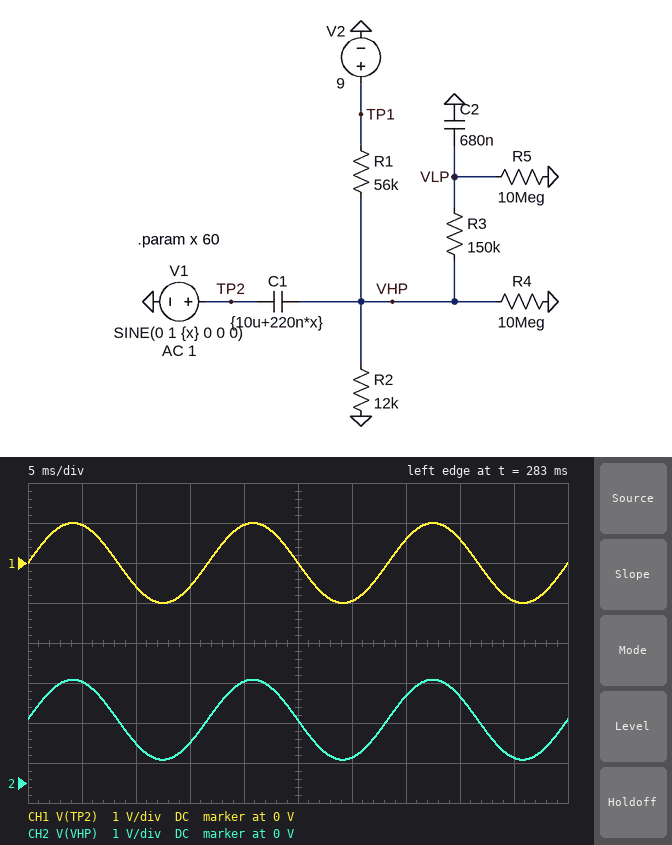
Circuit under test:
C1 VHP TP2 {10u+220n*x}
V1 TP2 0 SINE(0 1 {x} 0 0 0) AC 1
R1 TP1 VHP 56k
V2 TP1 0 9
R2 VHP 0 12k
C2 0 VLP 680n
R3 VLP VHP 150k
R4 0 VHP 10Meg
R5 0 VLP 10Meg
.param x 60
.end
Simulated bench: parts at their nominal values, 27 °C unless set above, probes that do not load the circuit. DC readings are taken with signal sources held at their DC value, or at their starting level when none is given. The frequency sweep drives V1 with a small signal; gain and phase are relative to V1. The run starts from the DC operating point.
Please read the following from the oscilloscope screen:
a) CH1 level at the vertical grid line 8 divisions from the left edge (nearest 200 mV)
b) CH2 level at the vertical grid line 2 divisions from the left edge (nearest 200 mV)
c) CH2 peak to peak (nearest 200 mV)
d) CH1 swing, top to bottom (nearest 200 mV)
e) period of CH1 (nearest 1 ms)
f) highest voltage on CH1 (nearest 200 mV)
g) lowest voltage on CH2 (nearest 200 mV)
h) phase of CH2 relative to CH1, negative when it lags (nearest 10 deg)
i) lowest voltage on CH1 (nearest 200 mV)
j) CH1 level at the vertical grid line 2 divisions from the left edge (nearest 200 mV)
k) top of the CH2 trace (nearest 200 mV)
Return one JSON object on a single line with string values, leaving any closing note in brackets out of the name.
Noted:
{"CH1 level at the vertical grid line 8 divisions from the left edge": "600 mV", "CH2 level at the vertical grid line 2 divisions from the left edge": "1.0 V", "CH2 peak to peak": "2.0 V", "CH1 swing, top to bottom": "2.0 V", "period of CH1": "17 ms", "highest voltage on CH1": "1.0 V", "lowest voltage on CH2": "600 mV", "phase of CH2 relative to CH1, negative when it lags": "0 deg", "lowest voltage on CH1": "-1.0 V", "CH1 level at the vertical grid line 2 divisions from the left edge": "-600 mV", "top of the CH2 trace": "2.6 V"}
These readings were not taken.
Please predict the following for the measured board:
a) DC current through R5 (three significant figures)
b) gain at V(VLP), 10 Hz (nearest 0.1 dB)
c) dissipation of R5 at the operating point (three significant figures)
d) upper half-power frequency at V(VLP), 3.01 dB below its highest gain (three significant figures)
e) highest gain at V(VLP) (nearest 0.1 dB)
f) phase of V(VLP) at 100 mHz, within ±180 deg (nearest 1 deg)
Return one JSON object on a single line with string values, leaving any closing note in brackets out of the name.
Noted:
{"DC current through R5": "156 nA", "gain at V(VLP), 10 Hz": "-16.3 dB", "dissipation of R5 at the operating point": "244 nW", "upper half-power frequency at V(VLP), 3.01 dB below its highest gain": "2.73 Hz", "highest gain at V(VLP)": "-3.5 dB", "phase of V(VLP) at 100 mHz, within ±180 deg": "78 deg"}
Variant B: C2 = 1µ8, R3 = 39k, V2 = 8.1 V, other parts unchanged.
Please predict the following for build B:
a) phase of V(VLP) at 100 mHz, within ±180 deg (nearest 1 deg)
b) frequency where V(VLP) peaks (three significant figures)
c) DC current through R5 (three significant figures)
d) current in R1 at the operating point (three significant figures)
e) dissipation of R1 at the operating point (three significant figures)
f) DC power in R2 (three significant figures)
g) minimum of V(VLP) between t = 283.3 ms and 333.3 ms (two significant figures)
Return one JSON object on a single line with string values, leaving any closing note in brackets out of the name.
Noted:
{"phase of V(VLP) at 100 mHz, within ±180 deg": "79 deg", "frequency where V(VLP) peaks": "1.26 Hz", "DC current through R5": "142 nA", "current in R1 at the operating point": "119 µA", "dissipation of R1 at the operating point": "795 µW", "DC power in R2": "170 µW", "minimum of V(VLP) between t = 283.3 ms and 333.3 ms": "1.4 V"}
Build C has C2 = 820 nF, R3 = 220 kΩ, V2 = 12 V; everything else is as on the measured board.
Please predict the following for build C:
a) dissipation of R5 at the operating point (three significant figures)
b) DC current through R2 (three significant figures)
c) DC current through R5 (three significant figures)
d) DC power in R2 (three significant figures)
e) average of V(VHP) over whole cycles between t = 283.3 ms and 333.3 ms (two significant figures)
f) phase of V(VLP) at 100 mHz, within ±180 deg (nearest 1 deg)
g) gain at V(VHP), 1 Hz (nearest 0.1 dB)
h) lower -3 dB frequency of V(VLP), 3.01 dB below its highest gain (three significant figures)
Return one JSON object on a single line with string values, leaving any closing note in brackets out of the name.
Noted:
{"dissipation of R5 at the operating point": "428 nW", "DC current through R2": "176 µA", "DC current through R5": "207 nA", "DC power in R2": "372 µW", "average of V(VHP) over whole cycles between t = 283.3 ms and 333.3 ms": "2.1 V", "phase of V(VLP) at 100 mHz, within ±180 deg": "75 deg", "gain at V(VHP), 1 Hz": "-1.9 dB", "lower -3 dB frequency of V(VLP), 3.01 dB below its highest gain": "322 mHz"}
